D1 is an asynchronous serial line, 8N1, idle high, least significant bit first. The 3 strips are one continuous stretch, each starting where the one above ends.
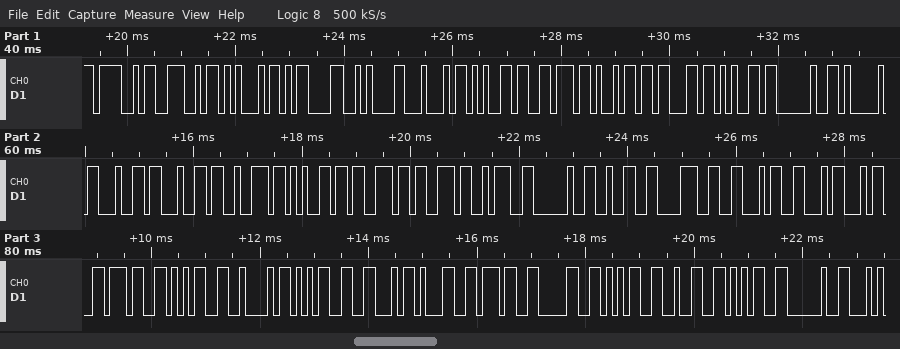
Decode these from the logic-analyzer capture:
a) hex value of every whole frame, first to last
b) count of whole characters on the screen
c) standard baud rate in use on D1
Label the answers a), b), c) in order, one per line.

a) 4F 4E 45 0D 0A 44 65 76 69 63 65 20 41 64 64 72 65 73 73 3A 20 32 38 46 46 34 37 35 42 35 46 31 37 30 35 32 35 20
b) 38
c) 9600 baud
